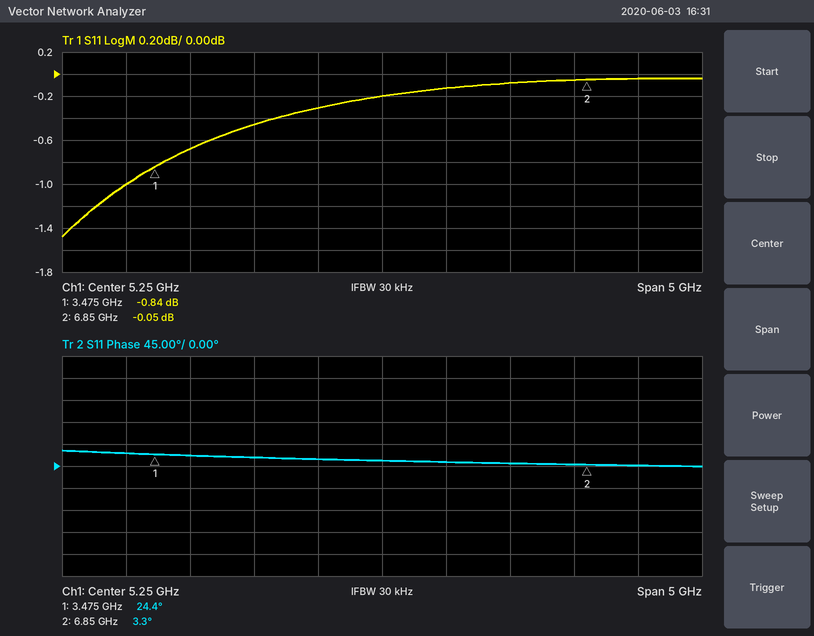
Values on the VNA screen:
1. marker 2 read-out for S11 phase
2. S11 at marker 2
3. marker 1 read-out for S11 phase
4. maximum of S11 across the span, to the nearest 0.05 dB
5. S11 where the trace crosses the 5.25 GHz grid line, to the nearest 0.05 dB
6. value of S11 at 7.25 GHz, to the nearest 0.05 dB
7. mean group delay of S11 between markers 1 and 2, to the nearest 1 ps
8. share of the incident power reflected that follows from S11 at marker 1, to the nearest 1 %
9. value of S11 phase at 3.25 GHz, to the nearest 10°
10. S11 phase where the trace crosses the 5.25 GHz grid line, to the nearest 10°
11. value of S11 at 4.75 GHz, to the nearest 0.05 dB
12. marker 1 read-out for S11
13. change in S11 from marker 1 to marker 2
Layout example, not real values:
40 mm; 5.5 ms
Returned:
3.3°; -0.05 dB; 24.4°; -0.05 dB; -0.20 dB; -0.05 dB; 17 ps; 82 %; 30°; 10°; -0.30 dB; -0.84 dB; 0.79 dB
